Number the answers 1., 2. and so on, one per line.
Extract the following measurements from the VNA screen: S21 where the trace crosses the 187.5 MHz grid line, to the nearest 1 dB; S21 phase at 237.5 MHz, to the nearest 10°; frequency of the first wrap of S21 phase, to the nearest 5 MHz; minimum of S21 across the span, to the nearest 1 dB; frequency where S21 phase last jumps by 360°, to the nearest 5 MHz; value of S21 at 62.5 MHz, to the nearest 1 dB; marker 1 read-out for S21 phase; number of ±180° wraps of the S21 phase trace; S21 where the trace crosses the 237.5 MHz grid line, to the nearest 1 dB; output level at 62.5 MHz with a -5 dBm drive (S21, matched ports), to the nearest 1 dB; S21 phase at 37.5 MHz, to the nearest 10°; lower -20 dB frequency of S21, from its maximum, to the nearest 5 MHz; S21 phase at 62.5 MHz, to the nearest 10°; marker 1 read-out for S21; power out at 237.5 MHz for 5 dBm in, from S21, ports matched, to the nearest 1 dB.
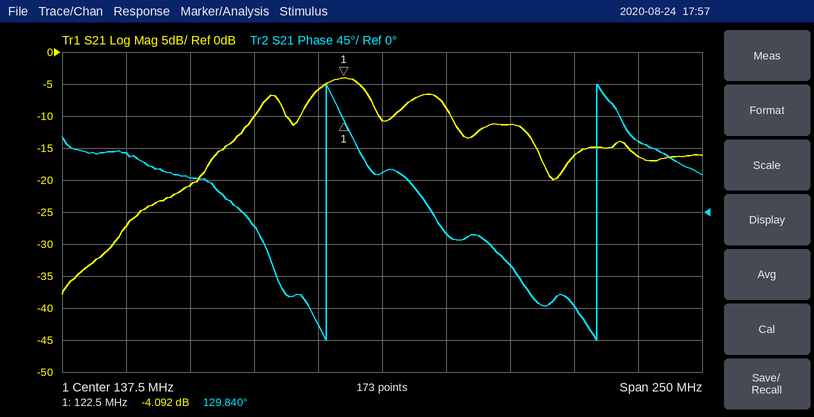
1. -11 dB
2. 100°
3. 115 MHz
4. -38 dB
5. 220 MHz
6. -21 dB
7. 129.840°
8. 2
9. -16 dB
10. -26 dBm
11. 80°
12. 45 MHz
13. 50°
14. -4.092 dB
15. -11 dBm
